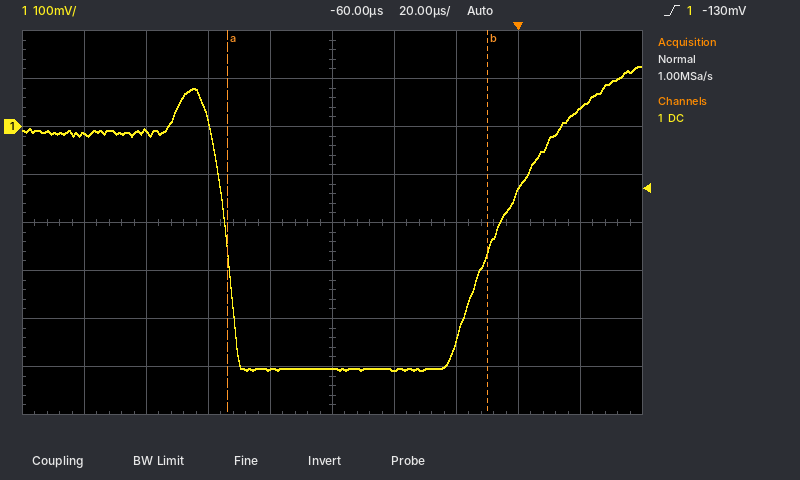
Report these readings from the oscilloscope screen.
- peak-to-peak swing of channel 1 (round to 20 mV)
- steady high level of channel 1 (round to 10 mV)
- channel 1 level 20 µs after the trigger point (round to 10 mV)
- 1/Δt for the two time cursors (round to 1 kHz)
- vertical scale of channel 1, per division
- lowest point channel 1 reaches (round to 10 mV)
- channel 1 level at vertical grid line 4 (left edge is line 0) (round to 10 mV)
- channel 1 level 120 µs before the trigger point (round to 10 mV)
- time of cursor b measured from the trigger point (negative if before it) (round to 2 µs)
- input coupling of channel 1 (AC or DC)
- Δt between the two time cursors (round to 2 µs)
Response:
640 mV
-10 mV
40 mV
12 kHz
100 mV
-510 mV
-510 mV
-10 mV
-10 µs
DC
84 µs
